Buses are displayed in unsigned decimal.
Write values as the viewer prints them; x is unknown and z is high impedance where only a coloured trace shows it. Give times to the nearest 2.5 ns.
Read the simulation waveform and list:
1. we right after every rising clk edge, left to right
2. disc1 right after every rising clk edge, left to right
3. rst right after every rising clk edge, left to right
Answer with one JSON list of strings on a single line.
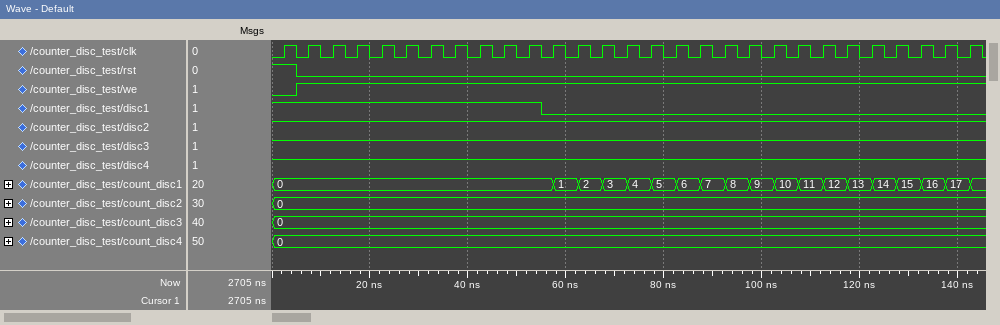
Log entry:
["0 1 1 1 1 1 1 1 1 1 1 1 1 1 1 1 1 1 1 1 1 1 1 1 1 1 1 1 1", "1 1 1 1 1 1 1 1 1 1 1 0 0 0 0 0 0 0 0 0 0 0 0 0 0 0 0 0 0", "1 0 0 0 0 0 0 0 0 0 0 0 0 0 0 0 0 0 0 0 0 0 0 0 0 0 0 0 0"]
